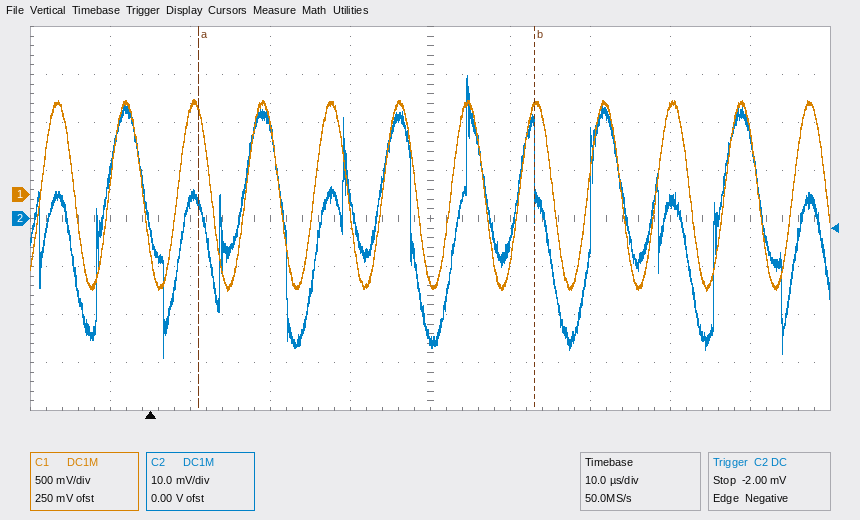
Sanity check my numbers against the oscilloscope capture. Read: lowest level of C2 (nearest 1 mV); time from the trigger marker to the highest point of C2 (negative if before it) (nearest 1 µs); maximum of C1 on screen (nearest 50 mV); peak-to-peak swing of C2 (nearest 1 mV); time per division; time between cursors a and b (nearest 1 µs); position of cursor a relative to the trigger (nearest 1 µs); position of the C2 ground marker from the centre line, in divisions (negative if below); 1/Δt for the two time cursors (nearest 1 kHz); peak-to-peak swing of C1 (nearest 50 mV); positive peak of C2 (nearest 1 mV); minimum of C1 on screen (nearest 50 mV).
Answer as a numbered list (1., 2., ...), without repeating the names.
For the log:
1. -29 mV
2. +40 µs
3. 1.00 V
4. 59 mV
5. 10 µs
6. 42 µs
7. +6 µs
8. 0.0 div
9. 24 kHz
10. 2.00 V
11. 30 mV
12. -1.00 V
